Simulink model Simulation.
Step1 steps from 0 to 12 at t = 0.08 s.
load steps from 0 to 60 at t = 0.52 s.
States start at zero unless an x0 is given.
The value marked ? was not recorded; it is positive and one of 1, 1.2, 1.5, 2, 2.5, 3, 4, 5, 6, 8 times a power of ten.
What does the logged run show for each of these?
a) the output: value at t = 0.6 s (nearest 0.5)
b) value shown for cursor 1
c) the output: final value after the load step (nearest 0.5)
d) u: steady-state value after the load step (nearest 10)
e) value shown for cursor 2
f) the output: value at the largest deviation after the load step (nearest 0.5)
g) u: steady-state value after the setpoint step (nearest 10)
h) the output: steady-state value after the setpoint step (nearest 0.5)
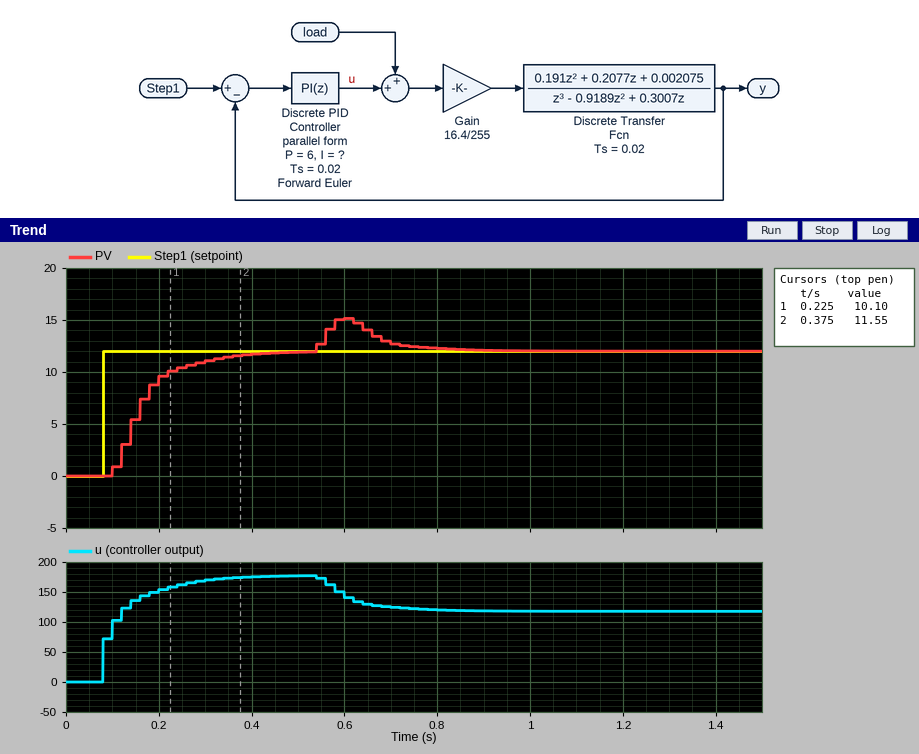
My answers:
15.0
10.10
12.0
120
11.55
15.0
180
12.0
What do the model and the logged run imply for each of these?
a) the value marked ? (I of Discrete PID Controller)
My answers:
150
